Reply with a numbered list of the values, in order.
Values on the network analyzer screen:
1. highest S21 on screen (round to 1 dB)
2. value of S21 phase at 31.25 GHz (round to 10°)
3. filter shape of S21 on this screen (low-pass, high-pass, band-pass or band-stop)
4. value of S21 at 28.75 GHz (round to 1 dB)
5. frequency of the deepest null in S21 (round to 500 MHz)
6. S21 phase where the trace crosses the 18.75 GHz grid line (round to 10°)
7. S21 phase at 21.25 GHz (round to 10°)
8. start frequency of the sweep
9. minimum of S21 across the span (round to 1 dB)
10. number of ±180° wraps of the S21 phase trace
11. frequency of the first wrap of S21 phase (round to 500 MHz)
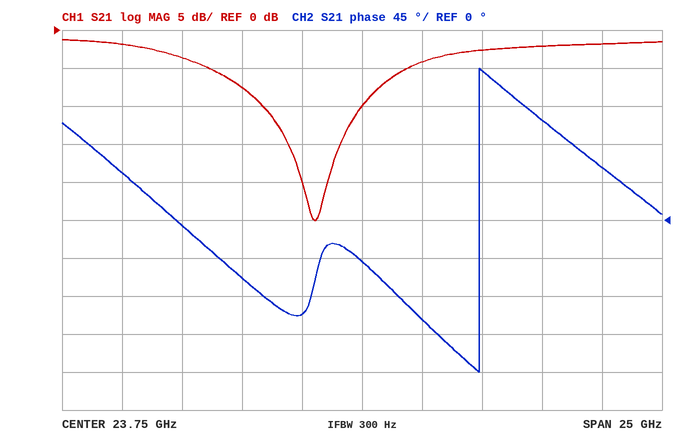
1. -1 dB
2. 120°
3. band-stop
4. -3 dB
5. 22.0 GHz
6. -70°
7. -110°
8. 11.25 GHz
9. -25 dB
10. 1
11. 28.5 GHz
